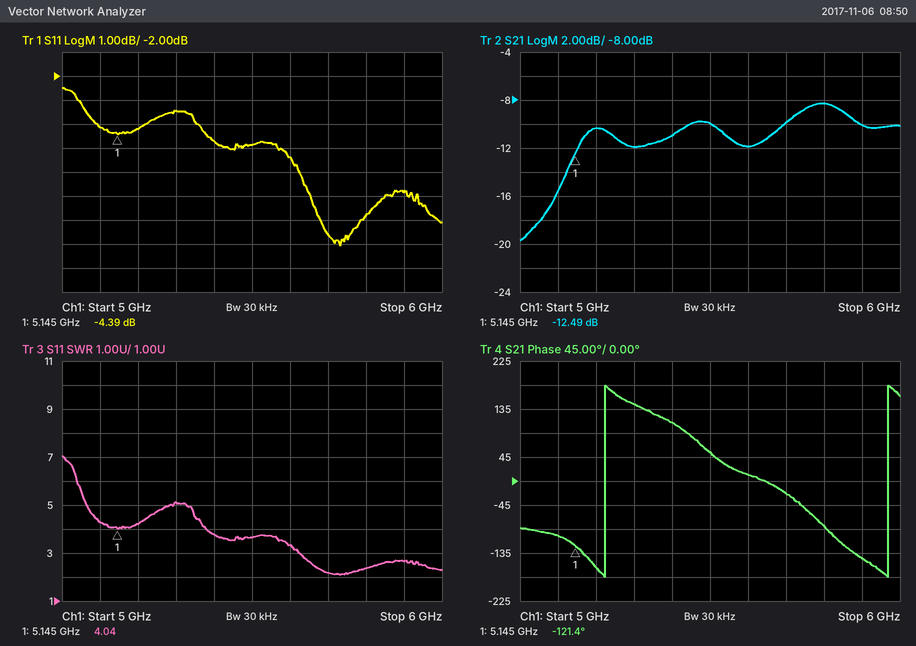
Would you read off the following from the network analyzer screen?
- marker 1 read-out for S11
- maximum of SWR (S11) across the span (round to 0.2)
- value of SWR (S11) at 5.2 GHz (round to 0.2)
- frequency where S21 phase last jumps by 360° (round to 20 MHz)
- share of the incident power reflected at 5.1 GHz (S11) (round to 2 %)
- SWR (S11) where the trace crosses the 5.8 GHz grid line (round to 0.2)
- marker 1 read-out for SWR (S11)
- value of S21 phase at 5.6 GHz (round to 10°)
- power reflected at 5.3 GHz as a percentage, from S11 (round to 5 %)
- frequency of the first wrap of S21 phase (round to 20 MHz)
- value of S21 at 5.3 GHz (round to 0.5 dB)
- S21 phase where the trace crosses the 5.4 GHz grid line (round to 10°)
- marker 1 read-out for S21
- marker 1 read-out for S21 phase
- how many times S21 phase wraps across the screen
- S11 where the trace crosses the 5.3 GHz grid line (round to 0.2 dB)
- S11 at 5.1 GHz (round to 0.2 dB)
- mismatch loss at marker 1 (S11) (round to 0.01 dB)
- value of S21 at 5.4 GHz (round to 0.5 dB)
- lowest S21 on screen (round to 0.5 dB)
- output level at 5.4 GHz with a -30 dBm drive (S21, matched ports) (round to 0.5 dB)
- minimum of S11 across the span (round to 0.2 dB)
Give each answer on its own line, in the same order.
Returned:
-4.39 dB
7.0
4.2
5.96 GHz
38 %
2.4
4.04
10°
45 %
5.22 GHz
-12.0 dB
110°
-12.49 dB
-121.4°
2
-3.4 dB
-4.2 dB
1.96 dB
-11.0 dB
-19.5 dB
-41.0 dBm
-9.0 dB
